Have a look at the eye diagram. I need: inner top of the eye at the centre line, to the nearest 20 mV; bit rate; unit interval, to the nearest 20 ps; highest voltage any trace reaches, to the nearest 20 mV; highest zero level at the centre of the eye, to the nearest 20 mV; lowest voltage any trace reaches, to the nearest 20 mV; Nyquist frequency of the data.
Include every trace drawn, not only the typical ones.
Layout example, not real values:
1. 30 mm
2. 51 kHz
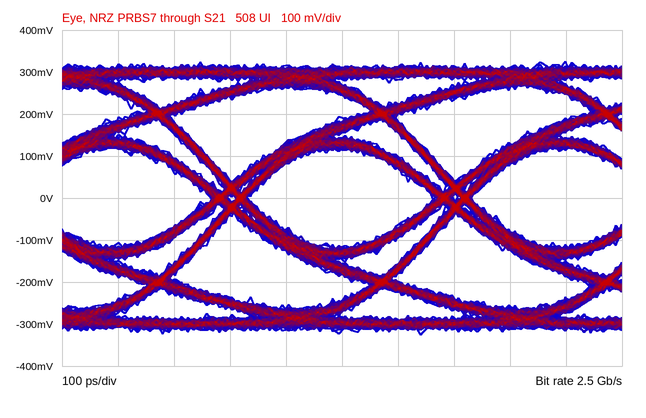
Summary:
1. 120 mV
2. 2.5 Gb/s
3. 400 ps
4. 320 mV
5. -120 mV
6. -320 mV
7. 1.25 GHz
